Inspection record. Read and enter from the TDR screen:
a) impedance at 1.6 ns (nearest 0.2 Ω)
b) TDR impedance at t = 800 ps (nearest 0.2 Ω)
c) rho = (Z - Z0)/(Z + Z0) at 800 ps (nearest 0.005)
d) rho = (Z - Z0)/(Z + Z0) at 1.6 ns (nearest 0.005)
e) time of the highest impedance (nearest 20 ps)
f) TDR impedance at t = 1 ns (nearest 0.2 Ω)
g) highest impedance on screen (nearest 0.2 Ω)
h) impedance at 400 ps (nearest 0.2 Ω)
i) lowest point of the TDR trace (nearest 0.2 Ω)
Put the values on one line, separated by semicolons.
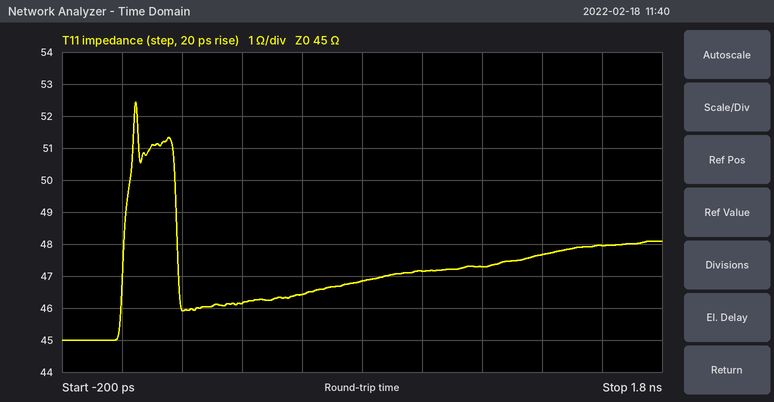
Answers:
48.0 Ω; 46.8 Ω; +0.020; +0.030; 40 ps; 47.2 Ω; 52.4 Ω; 46.2 Ω; 45.0 Ω
